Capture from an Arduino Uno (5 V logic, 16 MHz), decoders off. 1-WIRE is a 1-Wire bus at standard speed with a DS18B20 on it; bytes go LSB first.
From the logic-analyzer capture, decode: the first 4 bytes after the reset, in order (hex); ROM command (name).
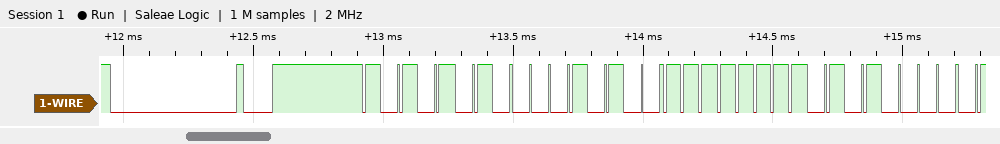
55 28 FF 0A
Match ROM
